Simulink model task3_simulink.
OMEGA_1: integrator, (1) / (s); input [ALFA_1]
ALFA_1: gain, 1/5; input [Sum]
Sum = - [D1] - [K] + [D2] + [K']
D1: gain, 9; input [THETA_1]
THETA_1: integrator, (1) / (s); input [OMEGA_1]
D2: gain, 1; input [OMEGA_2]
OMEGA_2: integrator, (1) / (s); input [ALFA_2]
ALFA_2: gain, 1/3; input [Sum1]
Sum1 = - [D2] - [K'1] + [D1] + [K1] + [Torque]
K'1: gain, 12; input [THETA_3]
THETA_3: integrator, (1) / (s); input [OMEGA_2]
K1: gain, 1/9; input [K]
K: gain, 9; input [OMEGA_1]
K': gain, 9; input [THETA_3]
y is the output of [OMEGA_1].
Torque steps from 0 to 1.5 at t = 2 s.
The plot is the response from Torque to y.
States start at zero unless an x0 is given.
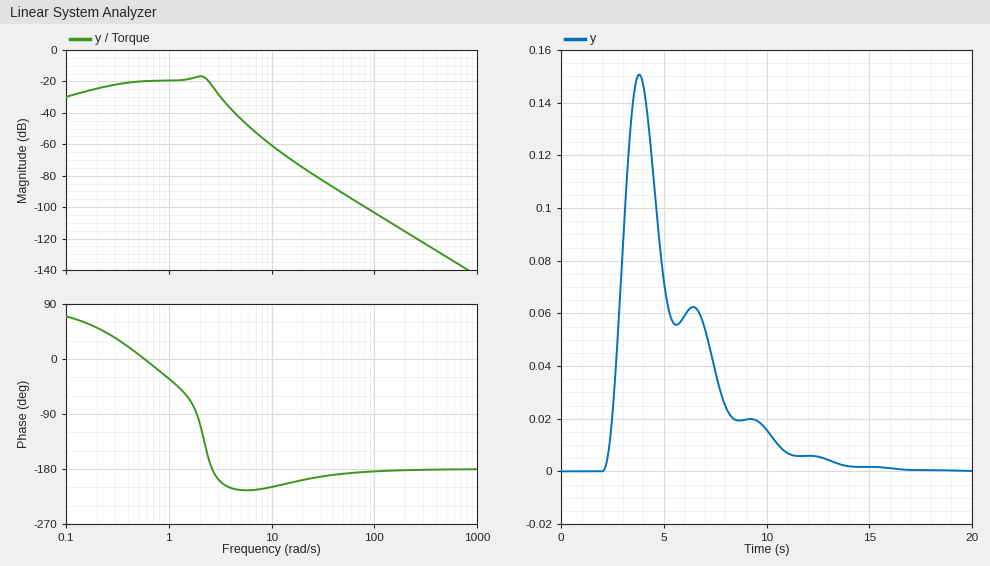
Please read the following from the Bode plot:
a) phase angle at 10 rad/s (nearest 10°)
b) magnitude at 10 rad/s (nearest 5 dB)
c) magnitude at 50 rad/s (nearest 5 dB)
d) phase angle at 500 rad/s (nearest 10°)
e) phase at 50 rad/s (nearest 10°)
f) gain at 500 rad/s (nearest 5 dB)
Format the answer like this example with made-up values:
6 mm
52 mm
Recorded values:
-210°
-60 dB
-90 dB
-180°
-190°
-130 dB
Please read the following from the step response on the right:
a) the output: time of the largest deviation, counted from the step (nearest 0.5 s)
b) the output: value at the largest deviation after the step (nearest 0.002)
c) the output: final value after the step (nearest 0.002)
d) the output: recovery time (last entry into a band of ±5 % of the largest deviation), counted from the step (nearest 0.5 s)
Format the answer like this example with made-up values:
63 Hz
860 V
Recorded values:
2.0 s
0.150
0.000
9.0 s
